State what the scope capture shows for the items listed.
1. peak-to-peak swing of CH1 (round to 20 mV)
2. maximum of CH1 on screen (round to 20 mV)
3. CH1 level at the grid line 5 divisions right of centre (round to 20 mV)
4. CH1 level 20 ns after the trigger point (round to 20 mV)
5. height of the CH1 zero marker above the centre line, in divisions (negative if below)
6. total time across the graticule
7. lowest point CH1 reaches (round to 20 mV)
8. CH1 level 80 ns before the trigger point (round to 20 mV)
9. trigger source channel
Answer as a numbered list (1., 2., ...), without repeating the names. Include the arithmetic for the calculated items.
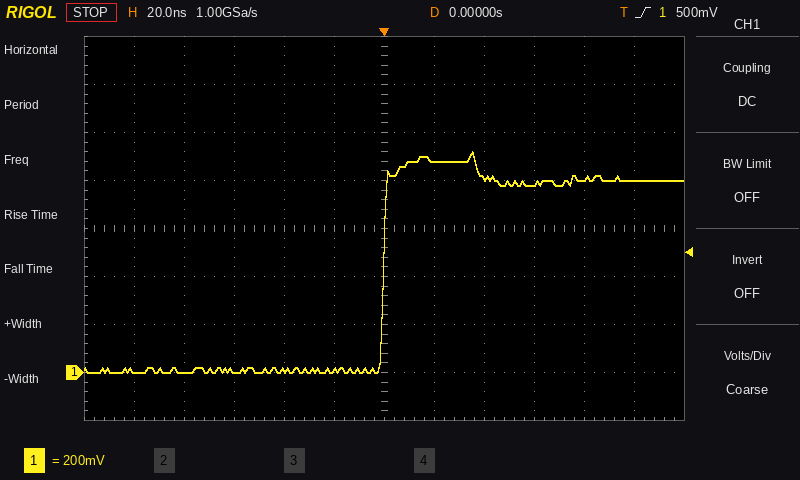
1. 920 mV − (0 mV) = 920 mV
2. 920 mV
3. 800 mV
4. 880 mV
5. -3.0 div
6. 240 ns
7. 0 mV
8. 0 mV
9. CH1
